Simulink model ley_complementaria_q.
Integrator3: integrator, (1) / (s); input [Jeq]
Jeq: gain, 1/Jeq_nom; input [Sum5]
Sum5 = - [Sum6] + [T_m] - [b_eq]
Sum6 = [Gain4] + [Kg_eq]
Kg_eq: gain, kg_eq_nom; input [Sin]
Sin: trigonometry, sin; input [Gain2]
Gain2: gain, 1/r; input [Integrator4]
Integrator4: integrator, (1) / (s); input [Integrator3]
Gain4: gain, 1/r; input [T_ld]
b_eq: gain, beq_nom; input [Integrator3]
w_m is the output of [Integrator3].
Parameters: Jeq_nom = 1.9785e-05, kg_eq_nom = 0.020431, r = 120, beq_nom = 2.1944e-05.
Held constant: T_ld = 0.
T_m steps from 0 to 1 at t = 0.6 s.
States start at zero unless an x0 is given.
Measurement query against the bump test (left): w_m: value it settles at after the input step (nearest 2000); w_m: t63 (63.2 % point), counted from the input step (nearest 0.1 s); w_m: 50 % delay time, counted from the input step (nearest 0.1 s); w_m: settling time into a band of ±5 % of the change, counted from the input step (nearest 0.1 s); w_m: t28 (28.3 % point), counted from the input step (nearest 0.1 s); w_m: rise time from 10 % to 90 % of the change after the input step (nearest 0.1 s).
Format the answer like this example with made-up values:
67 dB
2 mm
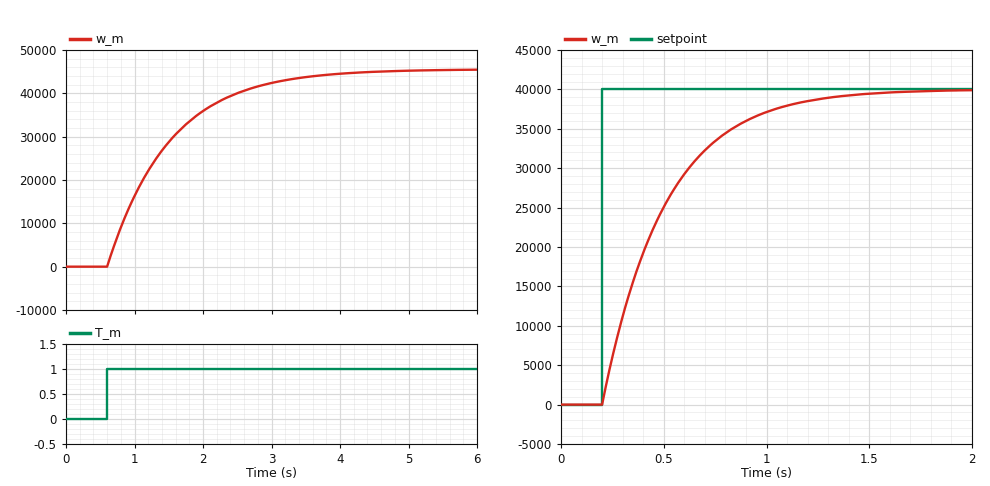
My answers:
46000
0.9 s
0.6 s
2.7 s
0.3 s
2.0 s
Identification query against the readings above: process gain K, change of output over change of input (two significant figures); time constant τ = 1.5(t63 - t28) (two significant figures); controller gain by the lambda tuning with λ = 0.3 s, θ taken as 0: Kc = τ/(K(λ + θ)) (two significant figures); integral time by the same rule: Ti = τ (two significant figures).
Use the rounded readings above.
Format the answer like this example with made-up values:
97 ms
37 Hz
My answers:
46000
0.90 s
0.000065
0.90 s
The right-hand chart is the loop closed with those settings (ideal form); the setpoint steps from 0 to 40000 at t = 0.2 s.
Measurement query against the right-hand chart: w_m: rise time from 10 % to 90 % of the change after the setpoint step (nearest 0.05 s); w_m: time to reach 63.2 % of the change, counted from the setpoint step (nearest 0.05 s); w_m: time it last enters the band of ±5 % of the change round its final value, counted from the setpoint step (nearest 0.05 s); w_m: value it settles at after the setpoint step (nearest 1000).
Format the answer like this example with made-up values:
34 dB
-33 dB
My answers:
0.65 s
0.30 s
0.90 s
40000
